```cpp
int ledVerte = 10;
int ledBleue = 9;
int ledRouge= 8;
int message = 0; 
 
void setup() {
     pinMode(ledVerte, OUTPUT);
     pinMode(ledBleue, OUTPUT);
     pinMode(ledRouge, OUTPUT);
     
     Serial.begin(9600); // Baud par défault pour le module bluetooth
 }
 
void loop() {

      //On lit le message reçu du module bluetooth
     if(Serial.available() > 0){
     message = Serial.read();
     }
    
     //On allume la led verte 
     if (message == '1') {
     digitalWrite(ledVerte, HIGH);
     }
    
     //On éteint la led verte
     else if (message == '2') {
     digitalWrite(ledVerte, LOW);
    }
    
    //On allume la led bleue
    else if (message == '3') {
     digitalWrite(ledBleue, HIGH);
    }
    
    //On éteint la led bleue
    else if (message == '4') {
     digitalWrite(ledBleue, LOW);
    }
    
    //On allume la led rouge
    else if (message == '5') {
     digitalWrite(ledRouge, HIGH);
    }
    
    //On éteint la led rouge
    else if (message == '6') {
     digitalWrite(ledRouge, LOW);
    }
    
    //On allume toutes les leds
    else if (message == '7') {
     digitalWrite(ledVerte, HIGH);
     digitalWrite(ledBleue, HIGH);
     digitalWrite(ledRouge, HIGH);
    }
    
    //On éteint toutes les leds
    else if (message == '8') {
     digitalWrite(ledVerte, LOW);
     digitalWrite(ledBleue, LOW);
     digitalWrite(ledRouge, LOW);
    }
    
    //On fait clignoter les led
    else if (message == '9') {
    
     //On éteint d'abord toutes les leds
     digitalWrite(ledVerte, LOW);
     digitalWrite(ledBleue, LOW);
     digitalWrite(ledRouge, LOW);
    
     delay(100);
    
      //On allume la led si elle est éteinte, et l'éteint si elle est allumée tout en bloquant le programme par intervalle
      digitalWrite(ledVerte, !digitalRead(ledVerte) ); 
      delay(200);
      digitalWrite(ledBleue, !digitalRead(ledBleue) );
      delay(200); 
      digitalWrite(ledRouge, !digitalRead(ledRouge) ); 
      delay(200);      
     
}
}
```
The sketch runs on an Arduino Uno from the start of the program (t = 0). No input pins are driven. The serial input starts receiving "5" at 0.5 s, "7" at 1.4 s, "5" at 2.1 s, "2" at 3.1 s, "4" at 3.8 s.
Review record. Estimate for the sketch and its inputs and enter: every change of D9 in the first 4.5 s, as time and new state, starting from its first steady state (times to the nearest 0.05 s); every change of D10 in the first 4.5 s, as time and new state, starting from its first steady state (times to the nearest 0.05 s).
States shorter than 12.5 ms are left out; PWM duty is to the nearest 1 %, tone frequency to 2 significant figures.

0 s low; 1.4 s high; 3.8 s low
0 s low; 1.4 s high; 3.1 s low
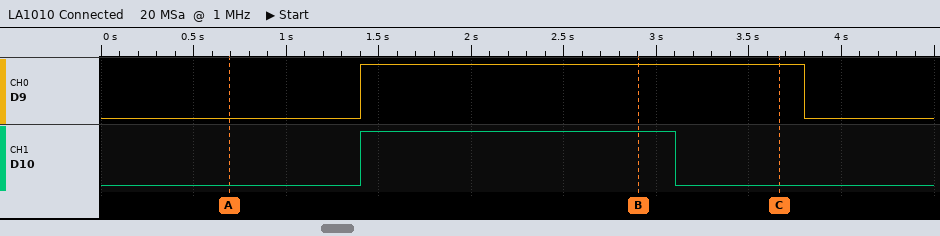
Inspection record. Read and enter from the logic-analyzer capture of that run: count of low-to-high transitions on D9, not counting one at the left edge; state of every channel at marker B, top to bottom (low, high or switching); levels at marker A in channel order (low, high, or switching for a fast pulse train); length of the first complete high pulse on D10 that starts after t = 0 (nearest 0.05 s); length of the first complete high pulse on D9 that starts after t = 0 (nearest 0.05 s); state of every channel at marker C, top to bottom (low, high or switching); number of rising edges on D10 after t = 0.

1
D9 high, D10 high
D9 low, D10 low
1.70 s
2.40 s
D9 high, D10 low
1
